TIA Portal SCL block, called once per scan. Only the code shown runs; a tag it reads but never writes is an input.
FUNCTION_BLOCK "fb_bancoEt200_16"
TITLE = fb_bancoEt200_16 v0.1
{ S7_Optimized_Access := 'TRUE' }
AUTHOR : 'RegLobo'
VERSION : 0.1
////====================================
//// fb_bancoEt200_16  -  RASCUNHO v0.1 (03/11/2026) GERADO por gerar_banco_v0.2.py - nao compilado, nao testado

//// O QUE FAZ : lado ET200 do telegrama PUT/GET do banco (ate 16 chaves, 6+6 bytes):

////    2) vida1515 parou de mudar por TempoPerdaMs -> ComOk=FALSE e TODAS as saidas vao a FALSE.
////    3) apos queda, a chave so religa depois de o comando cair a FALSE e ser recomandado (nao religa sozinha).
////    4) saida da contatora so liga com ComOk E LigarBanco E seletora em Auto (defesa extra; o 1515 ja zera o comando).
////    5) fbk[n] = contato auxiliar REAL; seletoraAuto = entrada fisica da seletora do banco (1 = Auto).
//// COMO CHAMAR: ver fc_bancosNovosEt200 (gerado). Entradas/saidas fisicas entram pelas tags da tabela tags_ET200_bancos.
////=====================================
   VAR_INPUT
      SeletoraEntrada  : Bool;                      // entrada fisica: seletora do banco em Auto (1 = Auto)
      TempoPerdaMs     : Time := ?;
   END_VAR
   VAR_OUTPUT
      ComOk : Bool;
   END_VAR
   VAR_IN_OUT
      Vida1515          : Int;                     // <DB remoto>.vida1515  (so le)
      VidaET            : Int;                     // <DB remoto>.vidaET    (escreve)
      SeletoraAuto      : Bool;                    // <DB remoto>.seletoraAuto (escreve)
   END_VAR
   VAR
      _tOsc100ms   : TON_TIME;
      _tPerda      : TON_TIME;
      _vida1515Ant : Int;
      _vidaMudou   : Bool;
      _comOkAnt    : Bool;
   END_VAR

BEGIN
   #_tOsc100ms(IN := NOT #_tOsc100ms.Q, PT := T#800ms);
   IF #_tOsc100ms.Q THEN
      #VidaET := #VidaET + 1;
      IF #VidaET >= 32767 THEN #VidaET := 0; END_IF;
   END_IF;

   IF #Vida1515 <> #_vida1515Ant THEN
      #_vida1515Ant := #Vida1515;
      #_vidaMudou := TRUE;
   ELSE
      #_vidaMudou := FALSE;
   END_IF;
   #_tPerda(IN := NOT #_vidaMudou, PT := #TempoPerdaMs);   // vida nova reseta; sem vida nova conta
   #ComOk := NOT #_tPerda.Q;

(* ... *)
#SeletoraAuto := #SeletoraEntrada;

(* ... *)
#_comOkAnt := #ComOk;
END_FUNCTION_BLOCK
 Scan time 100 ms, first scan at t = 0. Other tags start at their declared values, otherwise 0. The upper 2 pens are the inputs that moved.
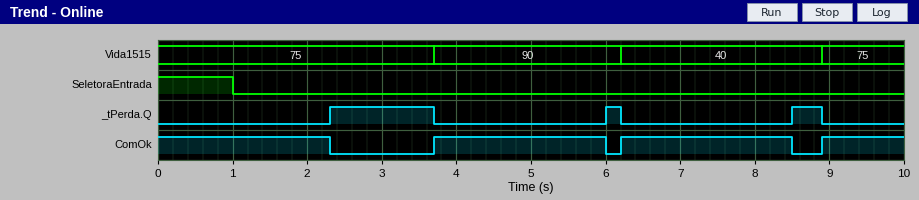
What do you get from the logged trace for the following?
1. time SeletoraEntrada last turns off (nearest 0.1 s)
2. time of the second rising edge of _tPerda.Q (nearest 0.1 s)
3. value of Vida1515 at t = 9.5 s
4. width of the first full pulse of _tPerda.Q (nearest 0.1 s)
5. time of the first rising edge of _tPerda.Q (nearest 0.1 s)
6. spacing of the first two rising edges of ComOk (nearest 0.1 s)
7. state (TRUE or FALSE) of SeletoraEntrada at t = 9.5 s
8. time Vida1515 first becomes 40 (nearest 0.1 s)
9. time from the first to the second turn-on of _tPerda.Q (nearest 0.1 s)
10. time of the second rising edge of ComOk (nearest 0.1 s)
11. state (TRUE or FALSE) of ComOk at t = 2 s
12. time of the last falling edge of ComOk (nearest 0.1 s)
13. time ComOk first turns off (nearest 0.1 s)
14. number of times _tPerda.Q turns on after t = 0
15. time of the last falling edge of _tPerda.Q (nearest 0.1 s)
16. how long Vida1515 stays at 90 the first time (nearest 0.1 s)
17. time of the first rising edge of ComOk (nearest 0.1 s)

1.0 s
6.0 s
75
1.4 s
2.3 s
2.5 s
FALSE
6.2 s
3.7 s
6.2 s
TRUE
8.5 s
2.3 s
3
8.9 s
2.5 s
3.7 s
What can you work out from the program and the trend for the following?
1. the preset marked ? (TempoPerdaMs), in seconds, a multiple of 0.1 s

2.2 s
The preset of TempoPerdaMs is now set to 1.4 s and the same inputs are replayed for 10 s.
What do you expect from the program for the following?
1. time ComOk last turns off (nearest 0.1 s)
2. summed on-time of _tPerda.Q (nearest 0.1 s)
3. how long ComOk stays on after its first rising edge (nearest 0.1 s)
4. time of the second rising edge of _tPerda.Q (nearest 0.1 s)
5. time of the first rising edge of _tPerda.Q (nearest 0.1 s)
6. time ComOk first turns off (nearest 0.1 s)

7.7 s
4.4 s
1.5 s
5.2 s
1.5 s
1.5 s
